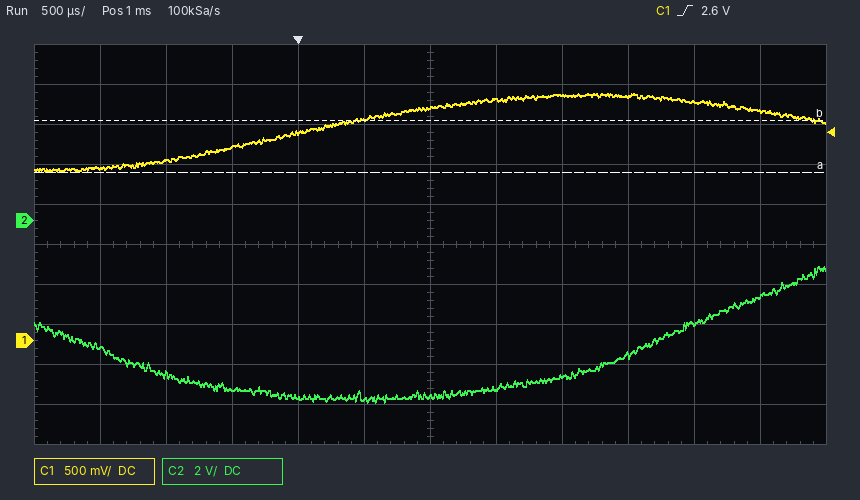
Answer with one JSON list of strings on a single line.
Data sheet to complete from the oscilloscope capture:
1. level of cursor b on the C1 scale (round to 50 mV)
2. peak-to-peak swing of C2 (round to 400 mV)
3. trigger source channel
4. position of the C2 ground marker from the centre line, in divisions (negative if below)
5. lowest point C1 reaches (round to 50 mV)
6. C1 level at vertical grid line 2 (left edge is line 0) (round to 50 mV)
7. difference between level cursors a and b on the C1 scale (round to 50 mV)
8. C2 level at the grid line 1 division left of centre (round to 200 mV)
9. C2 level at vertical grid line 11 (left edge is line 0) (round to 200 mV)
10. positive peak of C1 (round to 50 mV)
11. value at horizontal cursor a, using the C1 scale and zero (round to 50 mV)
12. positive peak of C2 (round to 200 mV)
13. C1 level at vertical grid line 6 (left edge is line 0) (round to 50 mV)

["2.75 V", "6.8 V", "C1", "+0.6 div", "2.10 V", "2.25 V", "650 mV", "-9.0 V", "-3.8 V", "3.10 V", "2.10 V", "-2.2 V", "2.90 V"]
